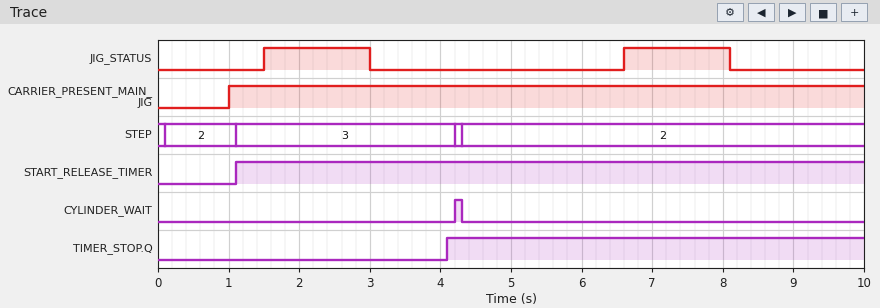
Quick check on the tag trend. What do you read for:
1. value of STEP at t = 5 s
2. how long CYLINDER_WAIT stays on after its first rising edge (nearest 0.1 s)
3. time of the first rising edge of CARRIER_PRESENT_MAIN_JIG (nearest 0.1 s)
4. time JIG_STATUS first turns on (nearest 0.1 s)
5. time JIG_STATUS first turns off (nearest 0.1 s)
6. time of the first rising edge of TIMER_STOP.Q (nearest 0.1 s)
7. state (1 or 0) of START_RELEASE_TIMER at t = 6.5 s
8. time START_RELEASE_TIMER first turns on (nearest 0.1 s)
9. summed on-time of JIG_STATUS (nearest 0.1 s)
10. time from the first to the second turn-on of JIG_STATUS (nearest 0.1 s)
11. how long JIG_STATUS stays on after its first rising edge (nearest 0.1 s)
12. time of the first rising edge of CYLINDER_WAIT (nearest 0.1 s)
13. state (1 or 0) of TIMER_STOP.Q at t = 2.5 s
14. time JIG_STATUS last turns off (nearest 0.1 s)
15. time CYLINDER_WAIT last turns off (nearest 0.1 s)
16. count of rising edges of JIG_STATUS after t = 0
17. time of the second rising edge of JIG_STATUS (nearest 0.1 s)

2
0.1 s
1.0 s
1.5 s
3.0 s
4.1 s
1
1.1 s
3.0 s
5.1 s
1.5 s
4.2 s
0
8.1 s
4.3 s
2
6.6 s
